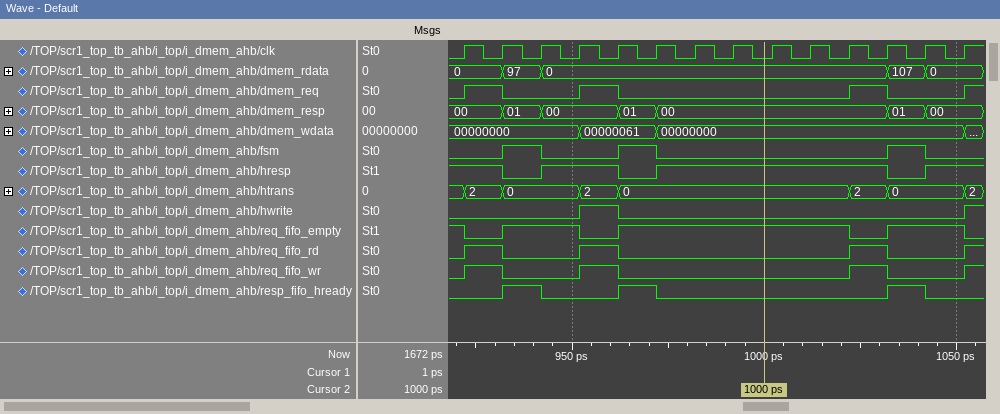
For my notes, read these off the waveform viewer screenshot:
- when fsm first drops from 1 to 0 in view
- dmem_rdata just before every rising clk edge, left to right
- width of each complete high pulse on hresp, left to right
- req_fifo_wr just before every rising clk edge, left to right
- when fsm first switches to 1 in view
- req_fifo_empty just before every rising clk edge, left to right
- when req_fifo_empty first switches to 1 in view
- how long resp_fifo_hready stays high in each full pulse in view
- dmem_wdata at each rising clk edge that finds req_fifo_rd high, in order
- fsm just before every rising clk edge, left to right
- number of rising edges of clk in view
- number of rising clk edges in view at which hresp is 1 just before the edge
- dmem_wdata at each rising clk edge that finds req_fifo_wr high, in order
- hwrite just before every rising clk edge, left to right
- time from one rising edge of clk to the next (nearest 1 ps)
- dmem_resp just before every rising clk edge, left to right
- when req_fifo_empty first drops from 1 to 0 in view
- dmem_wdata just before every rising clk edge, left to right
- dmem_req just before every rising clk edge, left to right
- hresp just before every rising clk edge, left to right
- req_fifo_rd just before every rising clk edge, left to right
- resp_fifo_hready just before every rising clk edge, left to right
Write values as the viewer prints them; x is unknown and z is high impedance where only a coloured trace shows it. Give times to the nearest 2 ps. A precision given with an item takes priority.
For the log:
942 ps
0, 0, 97, 0, 0, 0, 0, 0, 0, 0, 0, 0, 107, 0
20 ps, 60 ps
0 1 0 0 1 0 0 0 0 0 0 1 0 0
932 ps
1 0 1 1 0 1 1 1 1 1 1 0 1 1
932 ps
10 ps, 10 ps, 10 ps
00000000, 00000061, 00000000
0 0 1 0 0 1 0 0 0 0 0 0 1 0
14
11
00000000, 00000061, 00000000
0 0 0 0 1 0 0 0 0 0 0 0 0 0
10 ps
00, 00, 01, 00, 00, 01, 00, 00, 00, 00, 00, 00, 01, 00
922 ps
00000000, 00000000, 00000000, 00000000, 00000061, 00000061, 00000000, 00000000, 00000000, 00000000, 00000000, 00000000, 00000000, 00000000
0 1 0 0 1 0 0 0 0 0 0 1 0 0
1 1 0 1 1 0 1 1 1 1 1 1 0 1
0 1 0 0 1 0 0 0 0 0 0 1 0 0
0 0 1 0 0 1 0 0 0 0 0 0 1 0
